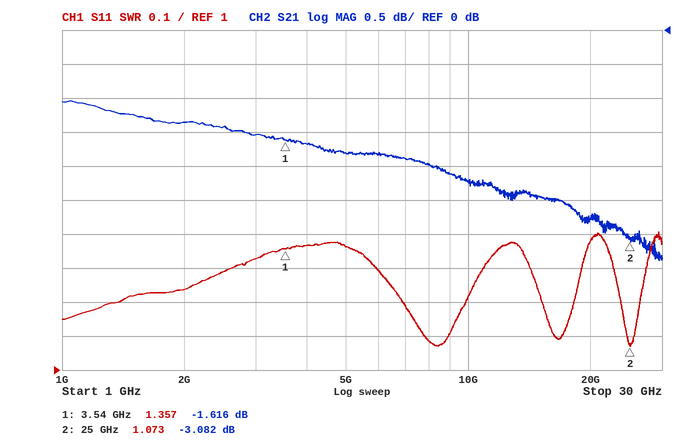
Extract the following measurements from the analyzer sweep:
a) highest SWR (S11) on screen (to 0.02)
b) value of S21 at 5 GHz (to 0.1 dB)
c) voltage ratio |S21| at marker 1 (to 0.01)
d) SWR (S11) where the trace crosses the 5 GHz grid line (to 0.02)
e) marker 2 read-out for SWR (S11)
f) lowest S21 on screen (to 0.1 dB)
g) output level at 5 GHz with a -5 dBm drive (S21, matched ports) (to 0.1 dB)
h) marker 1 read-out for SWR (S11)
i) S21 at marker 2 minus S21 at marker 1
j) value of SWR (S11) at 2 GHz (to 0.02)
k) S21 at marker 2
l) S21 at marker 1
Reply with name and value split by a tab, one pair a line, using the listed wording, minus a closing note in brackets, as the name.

highest SWR (S11) on screen	1.40
value of S21 at 5 GHz	-1.8 dB
voltage ratio |S21| at marker 1	0.83
SWR (S11) where the trace crosses the 5 GHz grid line	1.36
marker 2 read-out for SWR	1.073
lowest S21 on screen	-3.4 dB
output level at 5 GHz with a -5 dBm drive (S21, matched ports)	-6.8 dBm
marker 1 read-out for SWR	1.357
S21 at marker 2 minus S21 at marker 1	-1.466 dB
value of SWR (S11) at 2 GHz	1.24
S21 at marker 2	-3.082 dB
S21 at marker 1	-1.616 dB
